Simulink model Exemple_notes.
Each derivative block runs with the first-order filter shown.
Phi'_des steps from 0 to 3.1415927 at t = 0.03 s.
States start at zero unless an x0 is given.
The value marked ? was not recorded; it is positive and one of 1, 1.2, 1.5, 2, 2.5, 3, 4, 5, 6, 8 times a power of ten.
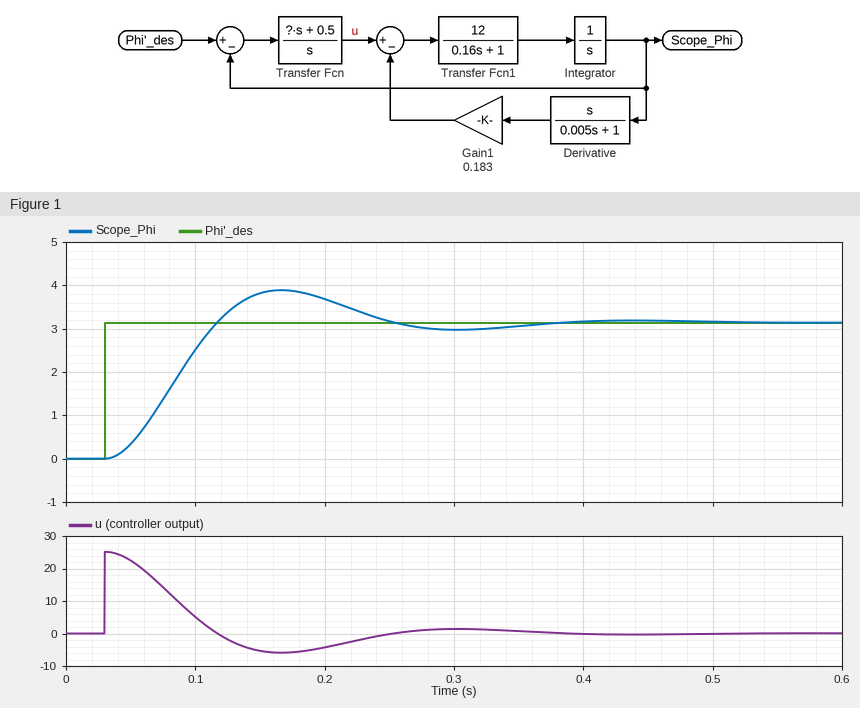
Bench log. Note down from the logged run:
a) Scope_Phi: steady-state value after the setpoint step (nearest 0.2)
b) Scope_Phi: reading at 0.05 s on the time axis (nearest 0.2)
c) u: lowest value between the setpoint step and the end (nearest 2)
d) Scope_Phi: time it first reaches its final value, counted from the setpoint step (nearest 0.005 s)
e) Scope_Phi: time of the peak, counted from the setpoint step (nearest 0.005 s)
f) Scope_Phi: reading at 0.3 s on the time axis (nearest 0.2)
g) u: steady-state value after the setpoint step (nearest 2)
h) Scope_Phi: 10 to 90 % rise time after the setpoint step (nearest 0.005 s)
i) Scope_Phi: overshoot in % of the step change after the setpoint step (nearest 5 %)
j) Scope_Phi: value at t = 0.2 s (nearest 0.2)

3.2
0.4
-6
0.085 s
0.135 s
3.0
0
0.060 s
25 %
3.6
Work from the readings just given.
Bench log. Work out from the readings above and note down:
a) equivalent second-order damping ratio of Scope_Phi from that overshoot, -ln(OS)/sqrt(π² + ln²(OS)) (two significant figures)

0.40
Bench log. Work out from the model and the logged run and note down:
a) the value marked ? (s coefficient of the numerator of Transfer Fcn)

8
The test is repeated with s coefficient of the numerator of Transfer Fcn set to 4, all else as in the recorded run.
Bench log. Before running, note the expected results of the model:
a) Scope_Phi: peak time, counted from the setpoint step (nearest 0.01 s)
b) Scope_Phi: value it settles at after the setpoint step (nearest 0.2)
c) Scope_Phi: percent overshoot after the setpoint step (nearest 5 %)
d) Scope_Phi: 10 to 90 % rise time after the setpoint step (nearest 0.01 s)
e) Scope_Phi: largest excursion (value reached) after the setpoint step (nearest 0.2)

0.22 s
3.2
10 %
0.10 s
3.4
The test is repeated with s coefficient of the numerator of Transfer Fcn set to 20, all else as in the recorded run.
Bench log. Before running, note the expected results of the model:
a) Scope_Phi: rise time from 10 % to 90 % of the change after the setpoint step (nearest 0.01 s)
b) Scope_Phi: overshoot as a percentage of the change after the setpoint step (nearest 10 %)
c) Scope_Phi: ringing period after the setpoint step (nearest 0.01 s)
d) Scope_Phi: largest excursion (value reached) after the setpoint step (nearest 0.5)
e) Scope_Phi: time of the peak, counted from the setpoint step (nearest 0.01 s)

0.03 s
40 %
0.16 s
4.5
0.08 s
